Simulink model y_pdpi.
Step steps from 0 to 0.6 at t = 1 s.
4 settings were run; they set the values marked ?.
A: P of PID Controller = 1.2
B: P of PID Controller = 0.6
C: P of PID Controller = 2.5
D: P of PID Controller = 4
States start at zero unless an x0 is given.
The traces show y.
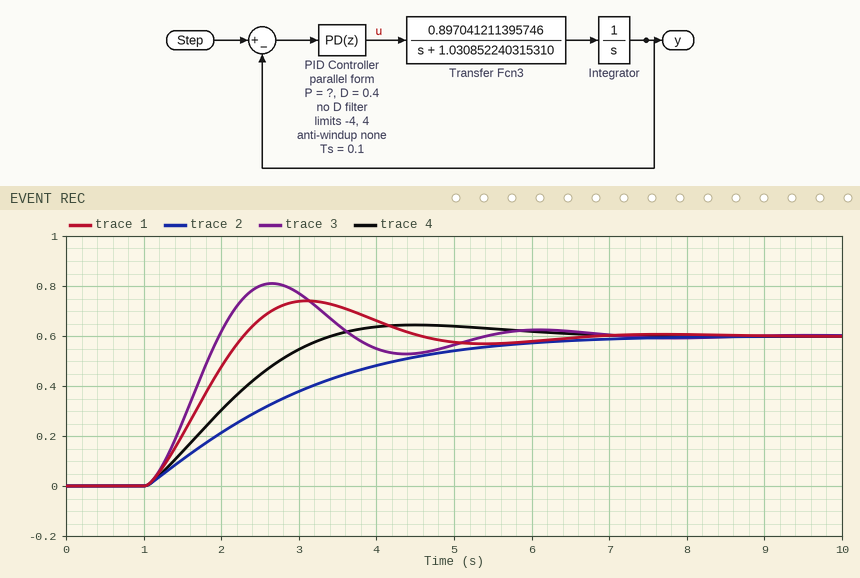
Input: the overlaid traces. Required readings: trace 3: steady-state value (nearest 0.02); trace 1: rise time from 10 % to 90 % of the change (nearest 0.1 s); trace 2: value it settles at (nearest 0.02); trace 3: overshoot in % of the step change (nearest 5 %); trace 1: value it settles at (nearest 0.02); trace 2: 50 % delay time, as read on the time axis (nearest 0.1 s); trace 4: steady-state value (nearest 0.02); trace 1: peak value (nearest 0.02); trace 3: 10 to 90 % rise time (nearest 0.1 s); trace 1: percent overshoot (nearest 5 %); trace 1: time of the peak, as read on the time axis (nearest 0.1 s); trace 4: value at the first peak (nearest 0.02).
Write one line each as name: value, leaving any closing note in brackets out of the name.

trace 3: steady-state value: 0.60
trace 1: rise time from 10 % to 90 % of the change: 0.9 s
trace 2: value it settles at: 0.60
trace 3: overshoot in % of the step change: 35 %
trace 1: value it settles at: 0.60
trace 2: 50 % delay time, as read on the time axis: 2.5 s
trace 4: steady-state value: 0.60
trace 1: peak value: 0.74
trace 3: 10 to 90 % rise time: 0.7 s
trace 1: percent overshoot: 25 %
trace 1: time of the peak, as read on the time axis: 3.1 s
trace 4: value at the first peak: 0.64
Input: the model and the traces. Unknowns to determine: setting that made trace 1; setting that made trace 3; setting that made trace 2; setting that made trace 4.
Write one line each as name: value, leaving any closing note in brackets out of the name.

setting that made trace 1: C
setting that made trace 3: D
setting that made trace 2: B
setting that made trace 4: A
